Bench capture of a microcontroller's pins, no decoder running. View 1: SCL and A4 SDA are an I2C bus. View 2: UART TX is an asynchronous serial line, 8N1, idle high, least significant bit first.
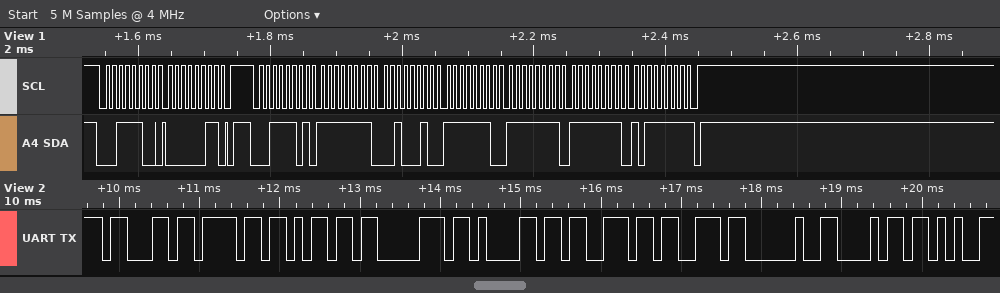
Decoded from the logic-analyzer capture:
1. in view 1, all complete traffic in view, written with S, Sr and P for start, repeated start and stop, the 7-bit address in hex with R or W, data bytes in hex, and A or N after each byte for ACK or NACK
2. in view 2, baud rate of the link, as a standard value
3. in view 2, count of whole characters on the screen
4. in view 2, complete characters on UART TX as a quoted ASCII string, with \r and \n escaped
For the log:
S 1EW A 03 A P S 1ER A FF A 22 A FE A FF A FF A BF N P
9600 baud
9
"compass h"
